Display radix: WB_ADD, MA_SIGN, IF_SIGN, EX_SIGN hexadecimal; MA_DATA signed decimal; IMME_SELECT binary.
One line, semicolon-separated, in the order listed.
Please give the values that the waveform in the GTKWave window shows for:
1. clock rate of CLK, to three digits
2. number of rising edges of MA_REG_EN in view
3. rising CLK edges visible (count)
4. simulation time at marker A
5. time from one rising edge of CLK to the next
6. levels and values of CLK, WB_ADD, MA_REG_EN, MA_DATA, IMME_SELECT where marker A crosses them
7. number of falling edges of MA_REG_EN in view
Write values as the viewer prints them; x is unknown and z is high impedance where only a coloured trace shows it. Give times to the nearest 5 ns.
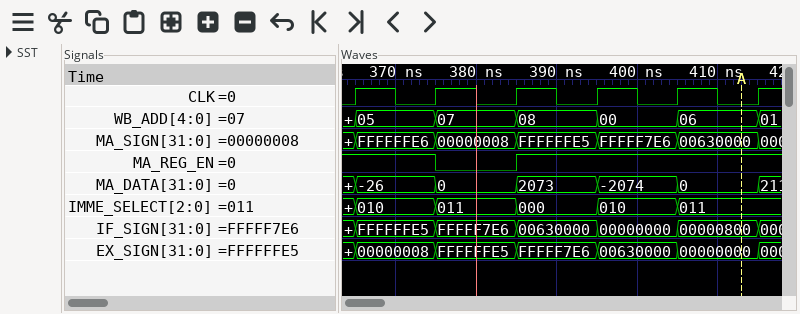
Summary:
100 MHz; 1; 6; 415 ns; 10 ns; CLK=0, WB_ADD=06, MA_REG_EN=1, MA_DATA=0, IMME_SELECT=011; 1
